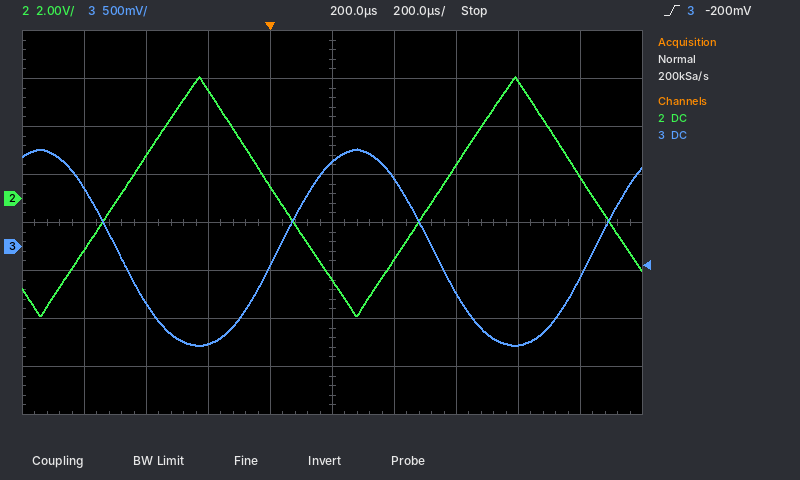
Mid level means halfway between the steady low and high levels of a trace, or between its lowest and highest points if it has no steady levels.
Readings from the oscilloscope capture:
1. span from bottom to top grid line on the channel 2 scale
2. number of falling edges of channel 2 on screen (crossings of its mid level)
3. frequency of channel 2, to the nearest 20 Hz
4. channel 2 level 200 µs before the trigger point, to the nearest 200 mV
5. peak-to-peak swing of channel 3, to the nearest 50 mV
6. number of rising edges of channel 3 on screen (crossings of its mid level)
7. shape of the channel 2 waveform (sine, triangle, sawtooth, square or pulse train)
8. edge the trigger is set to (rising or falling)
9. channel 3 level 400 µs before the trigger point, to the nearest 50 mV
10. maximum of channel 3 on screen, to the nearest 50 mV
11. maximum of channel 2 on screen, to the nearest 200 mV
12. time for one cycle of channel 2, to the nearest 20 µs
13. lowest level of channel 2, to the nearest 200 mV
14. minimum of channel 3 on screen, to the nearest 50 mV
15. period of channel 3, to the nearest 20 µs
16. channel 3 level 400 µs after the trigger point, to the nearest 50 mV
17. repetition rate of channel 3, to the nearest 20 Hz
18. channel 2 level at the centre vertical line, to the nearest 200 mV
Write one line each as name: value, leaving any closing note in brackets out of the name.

span from bottom to top grid line on the channel 2 scale: 16 V
number of falling edges of channel 2 on screen: 2
frequency of channel 2, to the nearest 20 Hz: 980 Hz
channel 2 level 200 µs before the trigger point, to the nearest 200 mV: 4.6 V
peak-to-peak swing of channel 3, to the nearest 50 mV: 2.05 V
number of rising edges of channel 3 on screen: 2
shape of the channel 2 waveform: triangle
edge the trigger is set to: rising
channel 3 level 400 µs before the trigger point, to the nearest 50 mV: -600 mV
maximum of channel 3 on screen, to the nearest 50 mV: 1.00 V
maximum of channel 2 on screen, to the nearest 200 mV: 5.0 V
time for one cycle of channel 2, to the nearest 20 µs: 1.02 ms
lowest level of channel 2, to the nearest 200 mV: -4.8 V
minimum of channel 3 on screen, to the nearest 50 mV: -1.05 V
period of channel 3, to the nearest 20 µs: 1.02 ms
channel 3 level 400 µs after the trigger point, to the nearest 50 mV: 700 mV
repetition rate of channel 3, to the nearest 20 Hz: 980 Hz
channel 2 level at the centre vertical line, to the nearest 200 mV: -3.4 V
